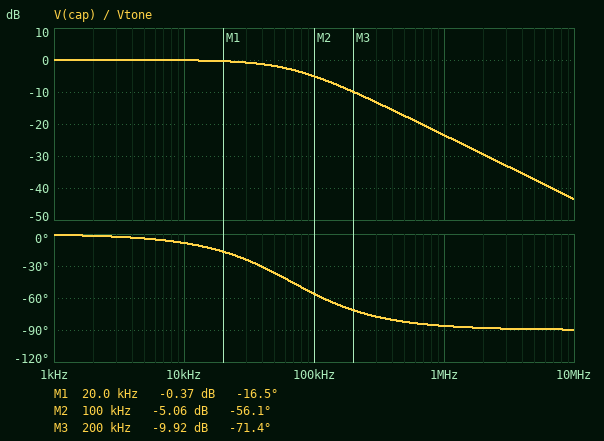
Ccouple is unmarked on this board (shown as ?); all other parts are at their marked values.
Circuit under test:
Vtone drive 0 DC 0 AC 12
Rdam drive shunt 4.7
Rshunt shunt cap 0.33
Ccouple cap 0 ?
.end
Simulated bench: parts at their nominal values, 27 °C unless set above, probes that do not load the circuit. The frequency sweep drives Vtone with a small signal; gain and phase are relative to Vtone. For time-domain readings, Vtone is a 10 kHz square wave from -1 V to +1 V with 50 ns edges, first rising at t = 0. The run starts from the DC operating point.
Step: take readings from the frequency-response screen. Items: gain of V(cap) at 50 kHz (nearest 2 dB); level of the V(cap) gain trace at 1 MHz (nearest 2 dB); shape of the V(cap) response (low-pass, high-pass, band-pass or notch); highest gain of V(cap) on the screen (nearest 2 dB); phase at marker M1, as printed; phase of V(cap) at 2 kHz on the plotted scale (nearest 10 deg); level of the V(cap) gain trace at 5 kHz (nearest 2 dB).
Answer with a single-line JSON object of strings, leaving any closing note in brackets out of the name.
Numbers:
{"gain of V(cap) at 50 kHz": "-2 dB", "level of the V(cap) gain trace at 1 MHz": "-24 dB", "shape of the V(cap) response": "low-pass", "highest gain of V(cap) on the screen": "0 dB", "phase at marker M1, as printed": "-16.5 deg", "phase of V(cap) at 2 kHz on the plotted scale": "0 deg", "level of the V(cap) gain trace at 5 kHz": "0 dB"}
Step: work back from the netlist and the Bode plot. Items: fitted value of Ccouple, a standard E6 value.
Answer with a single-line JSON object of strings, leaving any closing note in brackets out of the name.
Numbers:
{"fitted value of Ccouple, a standard E6 value": "470 nF"}
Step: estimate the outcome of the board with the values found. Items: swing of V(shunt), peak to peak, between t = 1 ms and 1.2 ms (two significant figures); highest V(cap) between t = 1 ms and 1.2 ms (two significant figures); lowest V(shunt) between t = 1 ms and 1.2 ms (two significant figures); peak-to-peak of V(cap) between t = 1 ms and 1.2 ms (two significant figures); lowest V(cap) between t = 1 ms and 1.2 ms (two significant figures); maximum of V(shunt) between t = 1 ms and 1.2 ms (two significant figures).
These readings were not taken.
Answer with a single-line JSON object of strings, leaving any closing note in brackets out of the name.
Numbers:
{"swing of V(shunt), peak to peak, between t = 1 ms and 1.2 ms": "2.0 V", "highest V(cap) between t = 1 ms and 1.2 ms": "1.0 V", "lowest V(shunt) between t = 1 ms and 1.2 ms": "-1.0 V", "peak-to-peak of V(cap) between t = 1 ms and 1.2 ms": "2.0 V", "lowest V(cap) between t = 1 ms and 1.2 ms": "-1.0 V", "maximum of V(shunt) between t = 1 ms and 1.2 ms": "1.0 V"}
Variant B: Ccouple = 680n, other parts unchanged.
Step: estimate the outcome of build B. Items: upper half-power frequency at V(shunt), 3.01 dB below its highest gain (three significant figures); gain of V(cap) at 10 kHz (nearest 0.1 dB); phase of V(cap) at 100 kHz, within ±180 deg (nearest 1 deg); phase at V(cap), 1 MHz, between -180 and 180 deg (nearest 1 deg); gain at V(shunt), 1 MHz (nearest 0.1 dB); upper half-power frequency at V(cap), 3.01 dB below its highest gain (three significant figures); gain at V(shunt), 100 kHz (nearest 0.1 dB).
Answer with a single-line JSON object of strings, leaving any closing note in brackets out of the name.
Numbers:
{"upper half-power frequency at V(shunt), 3.01 dB below its highest gain": "46.7 kHz", "gain of V(cap) at 10 kHz": "-0.2 dB", "phase of V(cap) at 100 kHz, within ±180 deg": "-65 deg", "phase at V(cap), 1 MHz, between -180 and 180 deg": "-87 deg", "gain at V(shunt), 1 MHz": "-21.9 dB", "upper half-power frequency at V(cap), 3.01 dB below its highest gain": "46.5 kHz", "gain at V(shunt), 100 kHz": "-7.4 dB"}
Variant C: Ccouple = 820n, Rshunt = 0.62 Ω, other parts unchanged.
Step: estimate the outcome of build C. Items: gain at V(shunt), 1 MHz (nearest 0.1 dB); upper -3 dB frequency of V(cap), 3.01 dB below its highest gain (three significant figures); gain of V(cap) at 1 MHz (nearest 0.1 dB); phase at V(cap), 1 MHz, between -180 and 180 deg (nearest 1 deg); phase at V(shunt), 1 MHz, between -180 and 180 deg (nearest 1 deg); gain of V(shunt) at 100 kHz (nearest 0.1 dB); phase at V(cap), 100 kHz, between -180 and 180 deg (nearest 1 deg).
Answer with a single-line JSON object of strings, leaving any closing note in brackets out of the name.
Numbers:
{"gain at V(shunt), 1 MHz": "-18.3 dB", "upper -3 dB frequency of V(cap), 3.01 dB below its highest gain": "36.5 kHz", "gain of V(cap) at 1 MHz": "-28.8 dB", "phase at V(cap), 1 MHz, between -180 and 180 deg": "-88 deg", "phase at V(shunt), 1 MHz, between -180 and 180 deg": "-15 deg", "gain of V(shunt) at 100 kHz": "-8.9 dB", "phase at V(cap), 100 kHz, between -180 and 180 deg": "-70 deg"}
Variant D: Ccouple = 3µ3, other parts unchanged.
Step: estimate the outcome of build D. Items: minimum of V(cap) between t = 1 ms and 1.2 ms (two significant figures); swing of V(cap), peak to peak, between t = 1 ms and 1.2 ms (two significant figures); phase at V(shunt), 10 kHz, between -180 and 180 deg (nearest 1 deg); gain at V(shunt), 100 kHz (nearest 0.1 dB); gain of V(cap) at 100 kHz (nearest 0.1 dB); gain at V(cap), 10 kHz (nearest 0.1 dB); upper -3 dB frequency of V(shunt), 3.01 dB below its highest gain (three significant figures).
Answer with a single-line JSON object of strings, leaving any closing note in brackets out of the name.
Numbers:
{"minimum of V(cap) between t = 1 ms and 1.2 ms": "-910 mV", "swing of V(cap), peak to peak, between t = 1 ms and 1.2 ms": "1.8 V", "phase at V(shunt), 10 kHz, between -180 and 180 deg": "-42 deg", "gain at V(shunt), 100 kHz": "-18.7 dB", "gain of V(cap) at 100 kHz": "-20.4 dB", "gain at V(cap), 10 kHz": "-3.2 dB", "upper -3 dB frequency of V(shunt), 3.01 dB below its highest gain": "9.63 kHz"}
